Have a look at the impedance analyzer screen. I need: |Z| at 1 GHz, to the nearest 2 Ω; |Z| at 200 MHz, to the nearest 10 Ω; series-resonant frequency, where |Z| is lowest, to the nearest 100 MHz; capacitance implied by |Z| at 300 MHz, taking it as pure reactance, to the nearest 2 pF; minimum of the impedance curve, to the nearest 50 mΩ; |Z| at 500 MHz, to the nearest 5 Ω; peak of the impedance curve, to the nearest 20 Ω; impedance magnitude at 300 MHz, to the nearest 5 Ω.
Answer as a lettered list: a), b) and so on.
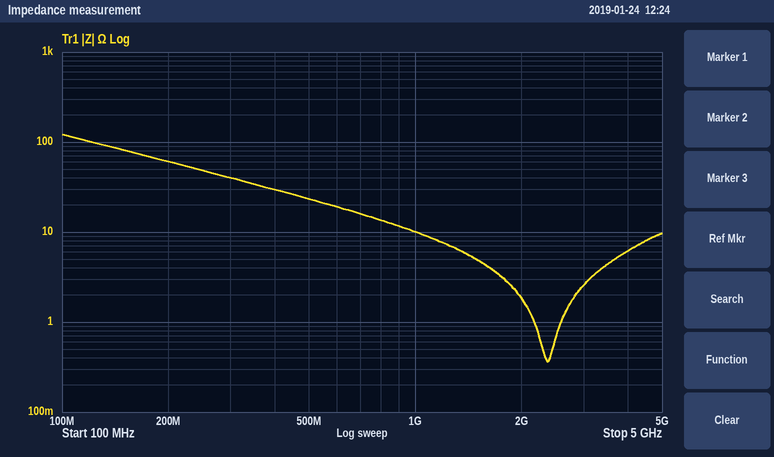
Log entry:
a) 10 Ω
b) 60 Ω
c) 2.4 GHz
d) 14 pF
e) 350 mΩ
f) 25 Ω
g) 120 Ω
h) 40 Ω
